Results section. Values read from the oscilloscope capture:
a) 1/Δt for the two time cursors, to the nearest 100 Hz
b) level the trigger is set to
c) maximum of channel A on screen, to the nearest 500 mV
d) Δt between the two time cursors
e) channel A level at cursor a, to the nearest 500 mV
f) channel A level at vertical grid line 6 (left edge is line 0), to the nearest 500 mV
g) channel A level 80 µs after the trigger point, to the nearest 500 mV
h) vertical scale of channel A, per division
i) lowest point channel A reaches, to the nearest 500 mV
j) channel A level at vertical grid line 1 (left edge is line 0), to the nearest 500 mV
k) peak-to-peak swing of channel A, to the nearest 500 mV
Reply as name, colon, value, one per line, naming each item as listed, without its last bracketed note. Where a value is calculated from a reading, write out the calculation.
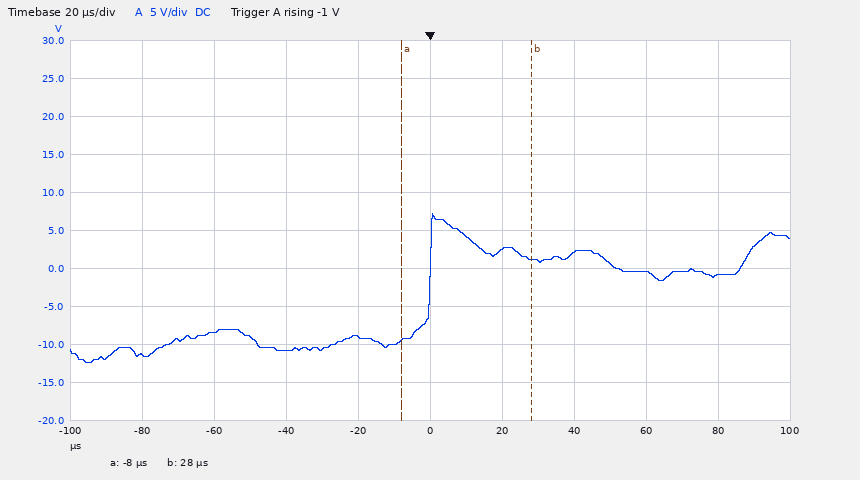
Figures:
1/Δt for the two time cursors, to the nearest 100 Hz: 1 / 36 µs ≈ 27.8 kHz
level the trigger is set to: -1 V
maximum of channel A on screen, to the nearest 500 mV: 7.0 V
Δt between the two time cursors: 28 µs − (-8 µs) = 36 µs
channel A level at cursor a, to the nearest 500 mV: -9.5 V
channel A level at vertical grid line 6 (left edge is line 0), to the nearest 500 mV: 2.5 V
channel A level 80 µs after the trigger point, to the nearest 500 mV: -1.0 V
vertical scale of channel A, per division: 5 V
lowest point channel A reaches, to the nearest 500 mV: -12.5 V
channel A level at vertical grid line 1 (left edge is line 0), to the nearest 500 mV: -11.5 V
peak-to-peak swing of channel A, to the nearest 500 mV: 7.0 V − (-12.5 V) = 19.5 V
